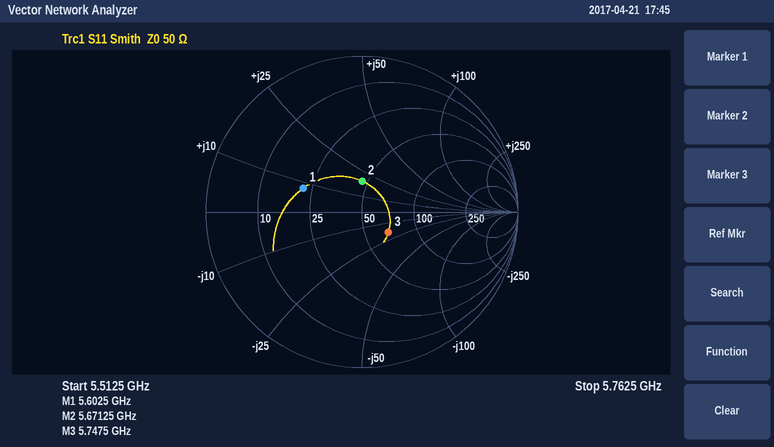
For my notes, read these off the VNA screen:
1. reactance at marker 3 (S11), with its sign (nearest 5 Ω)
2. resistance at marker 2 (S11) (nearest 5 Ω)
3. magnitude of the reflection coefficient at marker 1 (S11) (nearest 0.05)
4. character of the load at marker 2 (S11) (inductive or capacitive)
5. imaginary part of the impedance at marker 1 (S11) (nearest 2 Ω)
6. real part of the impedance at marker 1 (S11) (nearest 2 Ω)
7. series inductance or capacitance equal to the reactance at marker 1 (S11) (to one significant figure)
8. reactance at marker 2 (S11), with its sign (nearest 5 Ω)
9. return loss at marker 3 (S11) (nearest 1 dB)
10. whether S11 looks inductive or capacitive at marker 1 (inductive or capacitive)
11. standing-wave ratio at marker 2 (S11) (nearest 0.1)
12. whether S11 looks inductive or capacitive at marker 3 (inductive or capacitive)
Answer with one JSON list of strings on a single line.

["-20 Ω", "45 Ω", "0.40", "inductive", "+8 Ω", "22 Ω", "200 pH", "+20 Ω", "13 dB", "inductive", "1.5", "capacitive"]
